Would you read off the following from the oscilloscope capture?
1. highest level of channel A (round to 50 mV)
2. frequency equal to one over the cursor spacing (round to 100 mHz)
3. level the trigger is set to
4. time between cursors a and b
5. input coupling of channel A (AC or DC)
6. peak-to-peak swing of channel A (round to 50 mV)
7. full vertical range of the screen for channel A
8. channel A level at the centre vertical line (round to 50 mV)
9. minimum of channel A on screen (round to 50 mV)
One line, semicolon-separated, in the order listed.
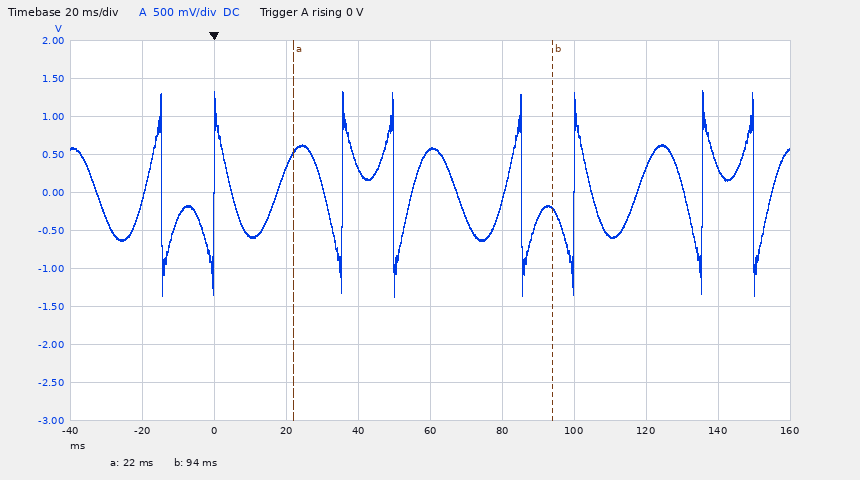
1.35 V; 13.9 Hz; 0 V; 72 ms; DC; 2.70 V; 5 V; 550 mV; -1.35 V
